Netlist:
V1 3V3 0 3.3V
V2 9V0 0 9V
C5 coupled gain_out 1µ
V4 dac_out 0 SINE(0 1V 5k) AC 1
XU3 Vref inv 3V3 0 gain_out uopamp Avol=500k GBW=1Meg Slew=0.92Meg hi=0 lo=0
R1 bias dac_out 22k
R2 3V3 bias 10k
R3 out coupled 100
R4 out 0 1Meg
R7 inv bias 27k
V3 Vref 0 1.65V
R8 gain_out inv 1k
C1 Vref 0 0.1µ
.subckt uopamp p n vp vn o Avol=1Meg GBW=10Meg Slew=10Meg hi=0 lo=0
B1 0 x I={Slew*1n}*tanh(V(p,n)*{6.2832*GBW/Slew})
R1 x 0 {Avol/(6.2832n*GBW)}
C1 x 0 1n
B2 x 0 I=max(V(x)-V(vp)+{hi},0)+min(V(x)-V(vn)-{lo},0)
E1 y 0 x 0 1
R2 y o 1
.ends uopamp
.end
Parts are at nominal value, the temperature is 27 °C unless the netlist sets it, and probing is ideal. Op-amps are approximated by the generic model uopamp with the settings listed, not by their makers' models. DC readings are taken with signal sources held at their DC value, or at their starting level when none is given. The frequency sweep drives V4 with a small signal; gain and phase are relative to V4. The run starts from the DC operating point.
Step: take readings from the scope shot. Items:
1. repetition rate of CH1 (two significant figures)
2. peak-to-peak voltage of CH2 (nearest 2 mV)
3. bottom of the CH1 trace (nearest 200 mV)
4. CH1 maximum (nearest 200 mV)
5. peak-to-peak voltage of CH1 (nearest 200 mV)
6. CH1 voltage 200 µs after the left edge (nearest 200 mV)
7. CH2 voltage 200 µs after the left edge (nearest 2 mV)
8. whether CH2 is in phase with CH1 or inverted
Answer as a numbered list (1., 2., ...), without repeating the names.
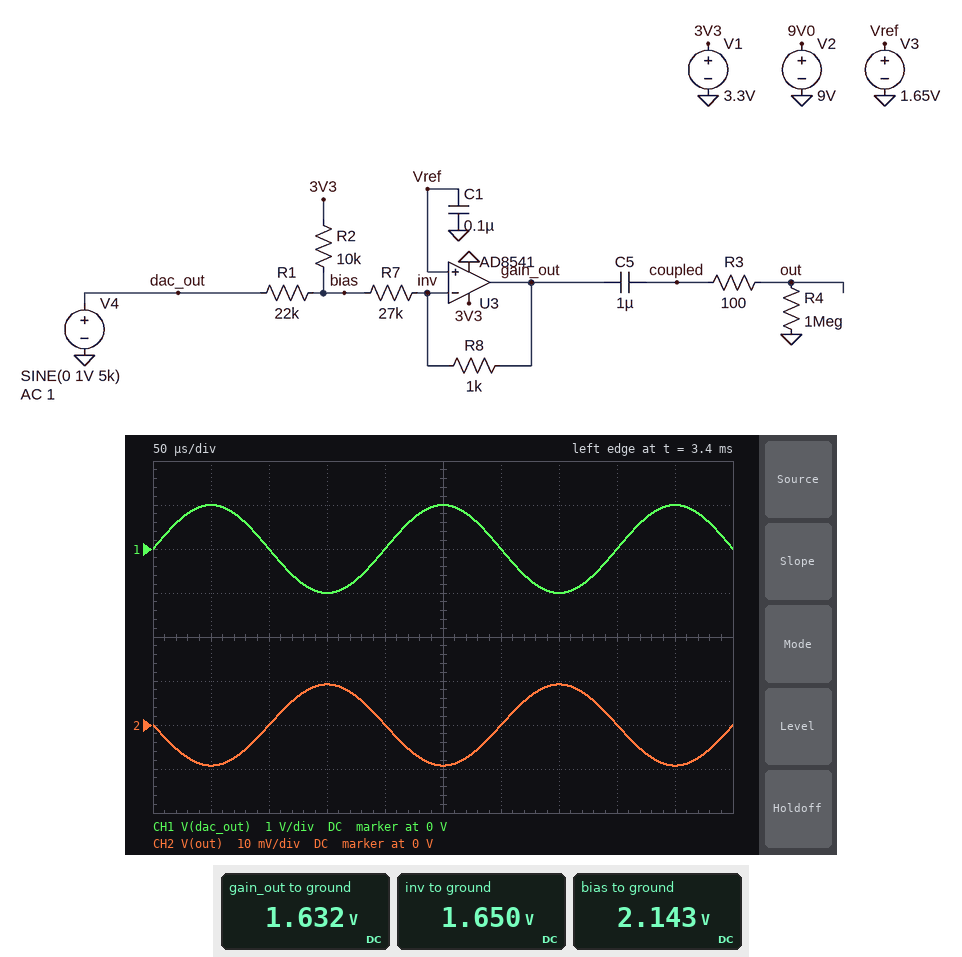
1. 5.0 kHz
2. 18 mV
3. -1.0 V
4. 1.0 V
5. 2.0 V
6. 0 V
7. 0 V
8. inverted
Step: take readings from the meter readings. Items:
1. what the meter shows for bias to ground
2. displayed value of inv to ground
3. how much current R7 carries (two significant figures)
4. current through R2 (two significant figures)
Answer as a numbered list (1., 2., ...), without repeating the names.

1. 2.143 V
2. 1.650 V
3. 18 µA
4. 120 µA
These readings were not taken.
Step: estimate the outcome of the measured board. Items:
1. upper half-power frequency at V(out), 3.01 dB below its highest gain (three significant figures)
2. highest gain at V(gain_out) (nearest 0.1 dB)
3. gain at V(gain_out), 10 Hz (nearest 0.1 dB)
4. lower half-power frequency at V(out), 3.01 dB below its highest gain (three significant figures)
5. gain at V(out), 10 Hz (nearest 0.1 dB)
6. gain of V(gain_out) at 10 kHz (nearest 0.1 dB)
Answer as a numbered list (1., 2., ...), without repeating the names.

1. 971 kHz
2. -40.7 dB
3. -40.7 dB
4. 159 mHz
5. -40.7 dB
6. -40.7 dB
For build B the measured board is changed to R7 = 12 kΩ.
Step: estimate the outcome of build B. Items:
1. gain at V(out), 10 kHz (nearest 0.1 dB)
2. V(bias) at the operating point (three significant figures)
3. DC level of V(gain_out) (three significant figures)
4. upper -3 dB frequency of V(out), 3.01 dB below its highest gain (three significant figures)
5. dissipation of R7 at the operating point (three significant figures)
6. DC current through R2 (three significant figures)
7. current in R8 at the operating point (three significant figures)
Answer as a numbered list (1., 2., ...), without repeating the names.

1. -35.6 dB
2. 2.04 V
3. 1.62 V
4. 950 kHz
5. 12.9 µW
6. 126 µA
7. 32.8 µA
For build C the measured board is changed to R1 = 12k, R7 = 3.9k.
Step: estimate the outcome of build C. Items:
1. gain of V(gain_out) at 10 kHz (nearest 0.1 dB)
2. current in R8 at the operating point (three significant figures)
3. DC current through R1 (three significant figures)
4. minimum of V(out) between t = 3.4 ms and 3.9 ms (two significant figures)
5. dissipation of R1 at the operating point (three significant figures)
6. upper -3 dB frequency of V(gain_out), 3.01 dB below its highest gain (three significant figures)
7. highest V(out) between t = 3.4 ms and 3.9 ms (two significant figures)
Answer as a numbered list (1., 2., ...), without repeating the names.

1. -26.3 dB
2. 16.0 µA
3. 143 µA
4. -49 mV
5. 244 µW
6. 903 kHz
7. 49 mV
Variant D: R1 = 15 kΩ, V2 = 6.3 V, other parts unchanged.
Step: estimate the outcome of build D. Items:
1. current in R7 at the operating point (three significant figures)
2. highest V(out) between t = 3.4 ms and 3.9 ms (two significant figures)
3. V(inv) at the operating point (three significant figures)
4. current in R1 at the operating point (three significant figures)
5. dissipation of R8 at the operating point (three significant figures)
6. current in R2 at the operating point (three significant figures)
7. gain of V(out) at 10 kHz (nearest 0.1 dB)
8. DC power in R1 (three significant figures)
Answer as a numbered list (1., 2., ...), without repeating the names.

1. 10.0 µA
2. 12 mV
3. 1.65 V
4. 128 µA
5. 100 nW
6. 138 µA
7. -38.3 dB
8. 246 µW
